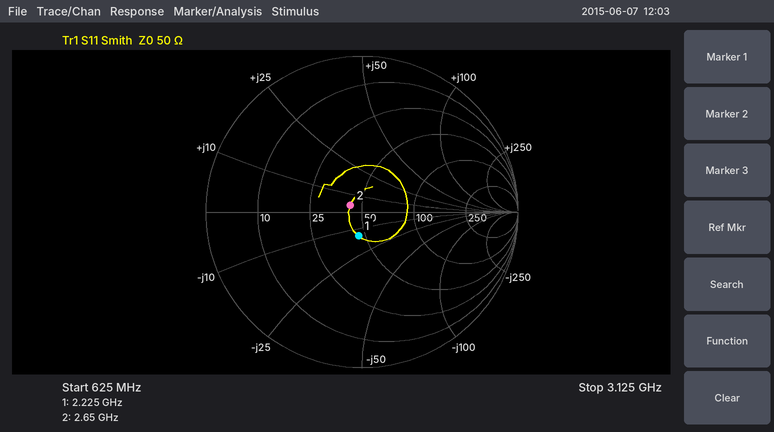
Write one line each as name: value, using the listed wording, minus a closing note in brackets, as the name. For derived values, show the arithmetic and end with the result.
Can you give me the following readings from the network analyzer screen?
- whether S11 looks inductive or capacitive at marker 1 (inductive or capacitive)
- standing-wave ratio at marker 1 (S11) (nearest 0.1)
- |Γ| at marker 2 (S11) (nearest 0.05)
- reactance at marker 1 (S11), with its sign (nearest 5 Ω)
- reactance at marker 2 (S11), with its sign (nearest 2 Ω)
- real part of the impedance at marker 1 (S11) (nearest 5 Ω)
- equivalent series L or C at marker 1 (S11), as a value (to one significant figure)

whether S11 looks inductive or capacitive at marker 1: capacitive
standing-wave ratio at marker 1 (S11): 1.4
|Γ| at marker 2 (S11): 0.10
reactance at marker 1 (S11), with its sign: -15 Ω
reactance at marker 2 (S11), with its sign: +4 Ω
real part of the impedance at marker 1 (S11): 45 Ω
equivalent series L or C at marker 1 (S11), as a value: C = 1/(2π × 2.225 GHz × 15 Ω) ≈ 5 pF
